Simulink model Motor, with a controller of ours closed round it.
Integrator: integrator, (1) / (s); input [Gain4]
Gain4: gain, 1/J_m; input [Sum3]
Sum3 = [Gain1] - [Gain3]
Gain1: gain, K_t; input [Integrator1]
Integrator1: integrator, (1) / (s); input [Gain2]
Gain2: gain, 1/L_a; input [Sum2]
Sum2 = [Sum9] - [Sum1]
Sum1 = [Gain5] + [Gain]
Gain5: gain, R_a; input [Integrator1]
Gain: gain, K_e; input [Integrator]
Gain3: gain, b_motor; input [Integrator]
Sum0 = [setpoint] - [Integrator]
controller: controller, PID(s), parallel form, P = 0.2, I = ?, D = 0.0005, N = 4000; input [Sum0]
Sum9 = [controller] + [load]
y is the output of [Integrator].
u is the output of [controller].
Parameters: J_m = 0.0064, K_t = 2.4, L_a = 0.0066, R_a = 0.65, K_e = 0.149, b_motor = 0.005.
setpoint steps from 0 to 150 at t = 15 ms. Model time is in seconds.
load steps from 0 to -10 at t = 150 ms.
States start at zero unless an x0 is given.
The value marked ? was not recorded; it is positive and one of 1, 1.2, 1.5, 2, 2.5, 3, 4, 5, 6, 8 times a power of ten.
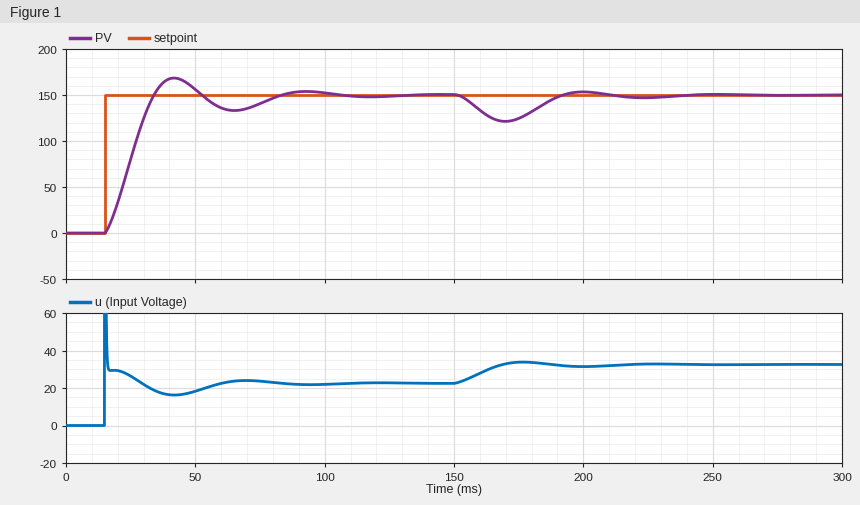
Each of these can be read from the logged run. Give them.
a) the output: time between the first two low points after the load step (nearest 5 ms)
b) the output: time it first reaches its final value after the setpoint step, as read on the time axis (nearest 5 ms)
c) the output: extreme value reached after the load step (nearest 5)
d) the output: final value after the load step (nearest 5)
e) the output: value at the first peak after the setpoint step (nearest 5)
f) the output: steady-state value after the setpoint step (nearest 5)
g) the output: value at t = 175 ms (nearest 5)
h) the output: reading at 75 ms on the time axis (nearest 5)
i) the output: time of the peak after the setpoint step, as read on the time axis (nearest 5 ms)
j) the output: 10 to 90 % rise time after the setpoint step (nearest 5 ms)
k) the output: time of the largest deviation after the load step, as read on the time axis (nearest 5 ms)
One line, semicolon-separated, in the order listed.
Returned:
55 ms; 35 ms; 120; 150; 170; 150; 125; 140; 40 ms; 15 ms; 170 ms
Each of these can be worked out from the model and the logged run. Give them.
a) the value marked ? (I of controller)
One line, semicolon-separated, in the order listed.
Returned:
15
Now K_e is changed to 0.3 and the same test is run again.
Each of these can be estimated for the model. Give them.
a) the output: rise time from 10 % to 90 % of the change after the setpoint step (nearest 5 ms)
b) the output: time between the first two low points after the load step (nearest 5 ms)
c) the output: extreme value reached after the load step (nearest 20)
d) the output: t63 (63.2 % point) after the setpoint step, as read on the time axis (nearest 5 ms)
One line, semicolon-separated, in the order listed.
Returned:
50 ms; 40 ms; 120; 30 ms
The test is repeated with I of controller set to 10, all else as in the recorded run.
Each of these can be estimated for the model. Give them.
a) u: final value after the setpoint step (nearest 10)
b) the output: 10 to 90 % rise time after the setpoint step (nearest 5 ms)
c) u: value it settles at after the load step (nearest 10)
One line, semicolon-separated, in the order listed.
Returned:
20; 15 ms; 30
